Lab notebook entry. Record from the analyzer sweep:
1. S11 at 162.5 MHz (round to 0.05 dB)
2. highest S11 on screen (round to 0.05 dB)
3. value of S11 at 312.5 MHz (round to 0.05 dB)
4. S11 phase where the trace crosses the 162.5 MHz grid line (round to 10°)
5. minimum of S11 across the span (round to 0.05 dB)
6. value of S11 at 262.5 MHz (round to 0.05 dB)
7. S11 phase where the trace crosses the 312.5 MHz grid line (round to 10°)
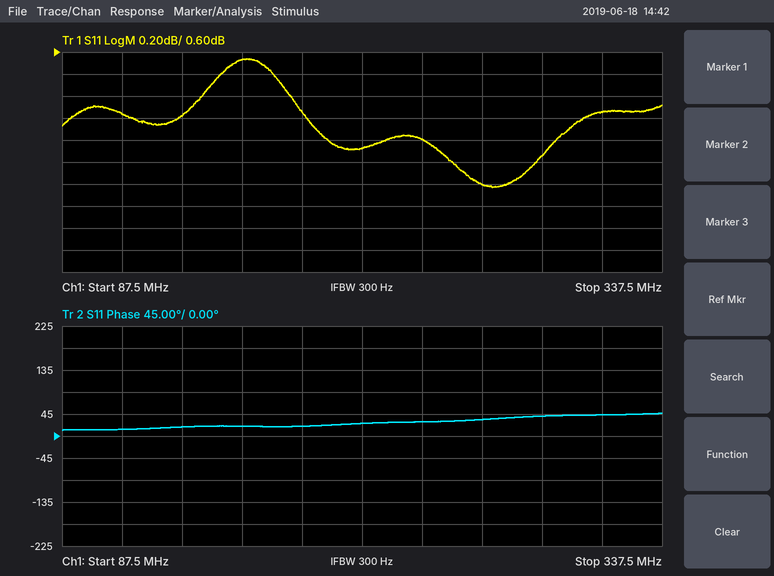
0.55 dB
0.55 dB
0.05 dB
20°
-0.65 dB
-0.60 dB
40°
